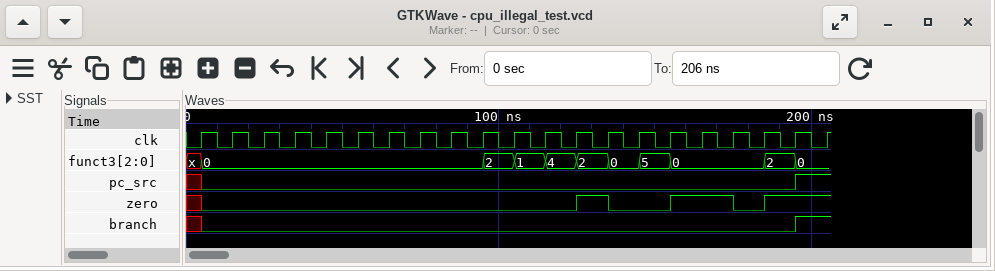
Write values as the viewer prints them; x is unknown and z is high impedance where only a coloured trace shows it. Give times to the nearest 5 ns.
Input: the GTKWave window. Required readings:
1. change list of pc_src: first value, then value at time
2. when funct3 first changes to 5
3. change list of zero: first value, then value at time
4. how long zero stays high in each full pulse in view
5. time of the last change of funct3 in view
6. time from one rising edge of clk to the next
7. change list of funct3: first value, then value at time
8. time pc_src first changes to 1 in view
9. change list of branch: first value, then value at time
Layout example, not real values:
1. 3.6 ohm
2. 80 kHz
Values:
1. x, 0 at 5 ns, 1 at 195 ns
2. 145 ns
3. x, 0 at 5 ns, 1 at 125 ns, 0 at 135 ns, 1 at 155 ns, 0 at 175 ns, 1 at 185 ns
4. 10 ns, 20 ns
5. 195 ns
6. 10 ns
7. x, 0 at 5 ns, 2 at 95 ns, 1 at 105 ns, 4 at 115 ns, 2 at 125 ns, 0 at 135 ns, 5 at 145 ns, 0 at 155 ns, 2 at 185 ns, 0 at 195 ns
8. 195 ns
9. x, 0 at 5 ns, 1 at 195 ns
